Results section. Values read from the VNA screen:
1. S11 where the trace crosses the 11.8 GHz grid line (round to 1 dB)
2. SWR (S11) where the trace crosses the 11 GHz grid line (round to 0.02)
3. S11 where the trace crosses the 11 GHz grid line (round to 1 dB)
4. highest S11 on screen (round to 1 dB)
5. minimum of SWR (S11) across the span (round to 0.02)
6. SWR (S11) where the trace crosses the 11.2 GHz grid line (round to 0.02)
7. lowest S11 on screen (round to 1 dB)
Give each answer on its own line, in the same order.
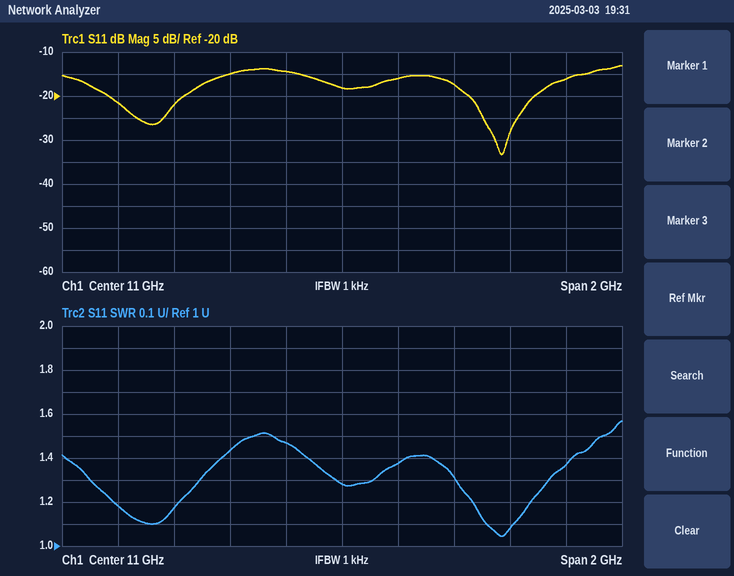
-16 dB
1.28
-18 dB
-13 dB
1.04
1.38
-33 dB
